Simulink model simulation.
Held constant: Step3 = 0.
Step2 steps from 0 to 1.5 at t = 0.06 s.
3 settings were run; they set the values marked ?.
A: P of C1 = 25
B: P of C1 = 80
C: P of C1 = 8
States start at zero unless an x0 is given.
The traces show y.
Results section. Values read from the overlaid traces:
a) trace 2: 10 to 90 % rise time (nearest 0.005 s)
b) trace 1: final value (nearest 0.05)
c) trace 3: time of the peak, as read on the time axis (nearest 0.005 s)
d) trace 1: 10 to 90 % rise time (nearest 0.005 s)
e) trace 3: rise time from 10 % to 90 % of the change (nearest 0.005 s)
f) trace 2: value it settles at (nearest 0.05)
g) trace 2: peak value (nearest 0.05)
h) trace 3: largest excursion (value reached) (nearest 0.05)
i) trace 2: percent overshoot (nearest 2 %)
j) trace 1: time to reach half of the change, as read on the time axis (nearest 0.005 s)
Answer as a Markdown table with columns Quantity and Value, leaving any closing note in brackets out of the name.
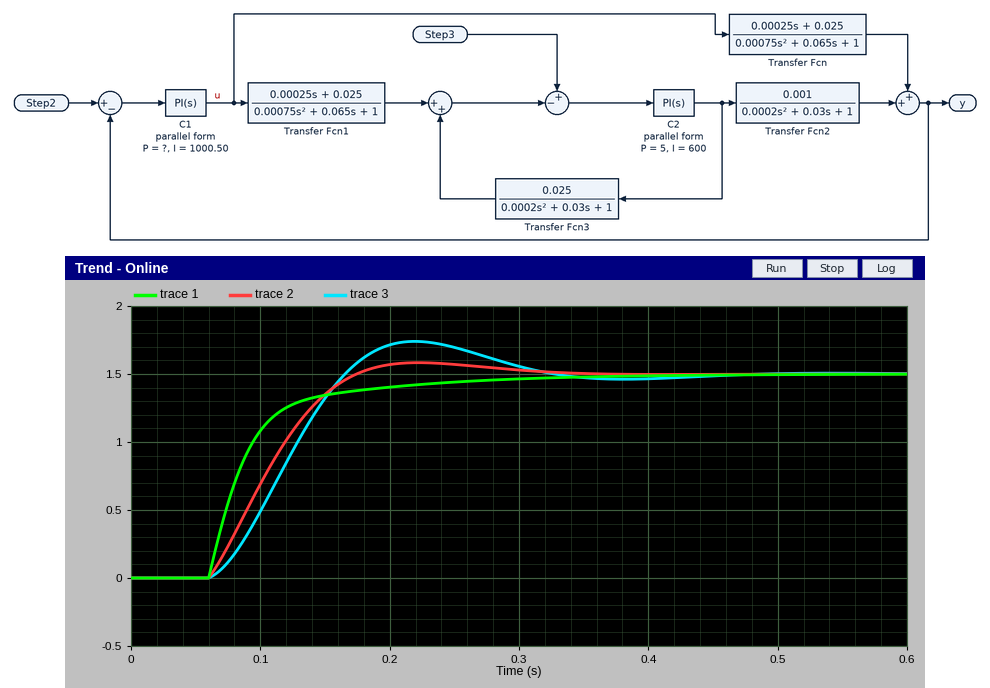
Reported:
| Quantity | Value |
|---|---|
| trace 2: 10 to 90 % rise time | 0.080 s |
| trace 1: final value | 1.50 |
| trace 3: time of the peak, as read on the time axis | 0.220 s |
| trace 1: 10 to 90 % rise time | 0.090 s |
| trace 3: rise time from 10 % to 90 % of the change | 0.075 s |
| trace 2: value it settles at | 1.50 |
| trace 2: peak value | 1.60 |
| trace 3: largest excursion (value reached) | 1.75 |
| trace 2: percent overshoot | 6 % |
| trace 1: time to reach half of the change, as read on the time axis | 0.080 s |
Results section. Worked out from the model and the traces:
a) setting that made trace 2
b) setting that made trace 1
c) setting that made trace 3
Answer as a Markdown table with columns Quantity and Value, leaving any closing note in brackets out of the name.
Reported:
| Quantity | Value |
|---|---|
| setting that made trace 2 | A |
| setting that made trace 1 | B |
| setting that made trace 3 | C |
